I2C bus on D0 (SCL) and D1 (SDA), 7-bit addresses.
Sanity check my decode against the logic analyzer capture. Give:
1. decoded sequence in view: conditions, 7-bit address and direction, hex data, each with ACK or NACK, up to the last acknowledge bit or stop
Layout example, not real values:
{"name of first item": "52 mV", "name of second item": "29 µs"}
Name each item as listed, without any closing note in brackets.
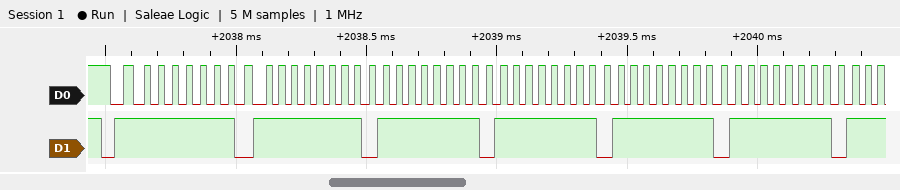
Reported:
{"decoded sequence in view: conditions, 7-bit address and direction, hex data, each with ACK or NACK, up to the last acknowledge bit or stop": "start, address 7F read ACK, FF ACK, FF ACK, FF ACK, FF ACK, FF ACK"}
